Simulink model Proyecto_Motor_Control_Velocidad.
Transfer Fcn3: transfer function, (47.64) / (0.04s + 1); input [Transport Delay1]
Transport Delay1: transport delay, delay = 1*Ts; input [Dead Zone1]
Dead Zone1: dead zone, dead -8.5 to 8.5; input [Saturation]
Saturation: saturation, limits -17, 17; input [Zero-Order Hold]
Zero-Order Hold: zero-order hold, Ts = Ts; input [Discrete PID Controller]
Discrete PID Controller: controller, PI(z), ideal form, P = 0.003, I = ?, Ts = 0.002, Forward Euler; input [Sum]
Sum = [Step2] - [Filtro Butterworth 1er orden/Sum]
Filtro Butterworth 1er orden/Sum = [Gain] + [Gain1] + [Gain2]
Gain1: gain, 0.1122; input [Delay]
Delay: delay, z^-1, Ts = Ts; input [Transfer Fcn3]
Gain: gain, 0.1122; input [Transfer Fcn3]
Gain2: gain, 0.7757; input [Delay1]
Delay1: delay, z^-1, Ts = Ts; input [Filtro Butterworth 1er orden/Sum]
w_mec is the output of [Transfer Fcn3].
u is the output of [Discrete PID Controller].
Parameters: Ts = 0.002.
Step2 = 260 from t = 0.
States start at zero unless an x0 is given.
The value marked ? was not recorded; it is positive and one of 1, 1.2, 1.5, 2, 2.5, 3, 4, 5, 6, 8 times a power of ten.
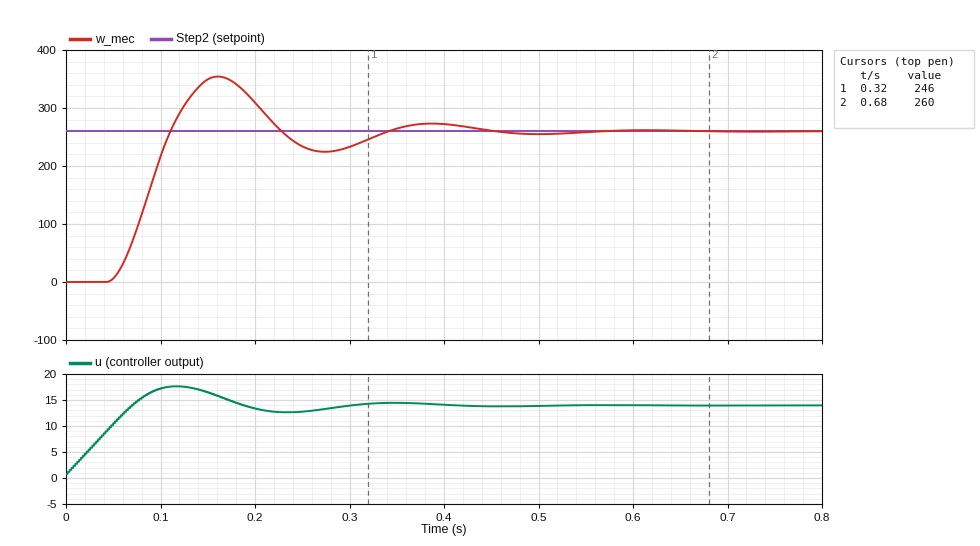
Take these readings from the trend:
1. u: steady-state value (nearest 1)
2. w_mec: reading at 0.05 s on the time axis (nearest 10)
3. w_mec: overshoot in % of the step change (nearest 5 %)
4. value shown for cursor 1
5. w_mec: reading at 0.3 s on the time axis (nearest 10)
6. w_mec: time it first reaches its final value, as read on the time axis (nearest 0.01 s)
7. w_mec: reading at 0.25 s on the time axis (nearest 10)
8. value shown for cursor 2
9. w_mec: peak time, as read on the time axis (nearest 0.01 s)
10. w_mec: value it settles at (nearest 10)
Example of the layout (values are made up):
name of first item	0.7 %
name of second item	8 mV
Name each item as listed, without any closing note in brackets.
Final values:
u: steady-state value	14
w_mec: reading at 0.05 s on the time axis	10
w_mec: overshoot in % of the step change	35 %
value shown for cursor 1	246
w_mec: reading at 0.3 s on the time axis	230
w_mec: time it first reaches its final value, as read on the time axis	0.11 s
w_mec: reading at 0.25 s on the time axis	230
value shown for cursor 2	260
w_mec: peak time, as read on the time axis	0.16 s
w_mec: value it settles at	260
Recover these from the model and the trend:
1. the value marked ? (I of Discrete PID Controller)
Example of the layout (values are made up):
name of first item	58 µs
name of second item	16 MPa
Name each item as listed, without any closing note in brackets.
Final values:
the value marked ?	250
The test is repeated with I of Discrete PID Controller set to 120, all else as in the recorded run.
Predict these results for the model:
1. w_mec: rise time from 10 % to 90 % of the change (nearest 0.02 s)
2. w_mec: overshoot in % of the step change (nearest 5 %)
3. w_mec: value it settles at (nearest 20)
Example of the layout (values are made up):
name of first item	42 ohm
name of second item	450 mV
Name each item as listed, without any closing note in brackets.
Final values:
w_mec: rise time from 10 % to 90 % of the change	0.08 s
w_mec: overshoot in % of the step change	10 %
w_mec: value it settles at	260
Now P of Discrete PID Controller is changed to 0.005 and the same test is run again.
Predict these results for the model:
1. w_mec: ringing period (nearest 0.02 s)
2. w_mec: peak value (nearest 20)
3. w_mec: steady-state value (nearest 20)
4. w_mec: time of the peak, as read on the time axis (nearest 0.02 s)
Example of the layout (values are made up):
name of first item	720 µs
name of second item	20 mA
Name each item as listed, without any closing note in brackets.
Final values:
w_mec: ringing period	0.18 s
w_mec: peak value	380
w_mec: steady-state value	260
w_mec: time of the peak, as read on the time axis	0.14 s
